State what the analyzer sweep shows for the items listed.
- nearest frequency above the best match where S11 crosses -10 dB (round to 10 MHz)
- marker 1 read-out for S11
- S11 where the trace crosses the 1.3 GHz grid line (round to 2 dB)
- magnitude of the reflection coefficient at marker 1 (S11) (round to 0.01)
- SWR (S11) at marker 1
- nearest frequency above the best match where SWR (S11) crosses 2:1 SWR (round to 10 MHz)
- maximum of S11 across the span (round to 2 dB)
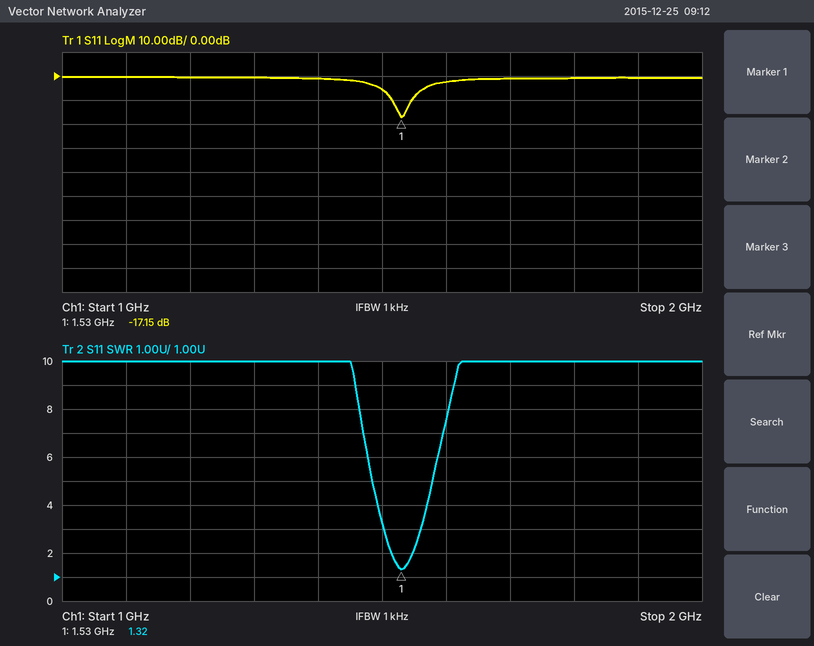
1.55 GHz
-17.15 dB
0 dB
0.14
1.32
1.55 GHz
0 dB
